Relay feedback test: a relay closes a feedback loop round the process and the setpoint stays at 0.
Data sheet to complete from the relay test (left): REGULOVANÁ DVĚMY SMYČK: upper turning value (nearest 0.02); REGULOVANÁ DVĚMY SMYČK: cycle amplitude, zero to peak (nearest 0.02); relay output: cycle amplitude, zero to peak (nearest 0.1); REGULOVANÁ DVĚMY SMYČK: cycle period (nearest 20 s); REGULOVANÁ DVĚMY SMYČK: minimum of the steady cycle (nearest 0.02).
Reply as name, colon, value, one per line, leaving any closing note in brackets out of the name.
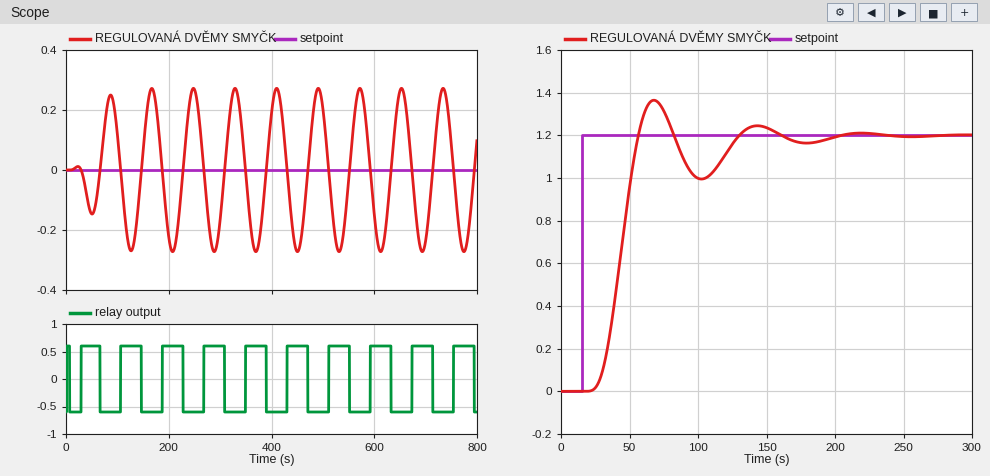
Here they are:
REGULOVANÁ DVĚMY SMYČK: upper turning value: 0.28
REGULOVANÁ DVĚMY SMYČK: cycle amplitude, zero to peak: 0.28
relay output: cycle amplitude, zero to peak: 0.6
REGULOVANÁ DVĚMY SMYČK: cycle period: 80 s
REGULOVANÁ DVĚMY SMYČK: minimum of the steady cycle: -0.28
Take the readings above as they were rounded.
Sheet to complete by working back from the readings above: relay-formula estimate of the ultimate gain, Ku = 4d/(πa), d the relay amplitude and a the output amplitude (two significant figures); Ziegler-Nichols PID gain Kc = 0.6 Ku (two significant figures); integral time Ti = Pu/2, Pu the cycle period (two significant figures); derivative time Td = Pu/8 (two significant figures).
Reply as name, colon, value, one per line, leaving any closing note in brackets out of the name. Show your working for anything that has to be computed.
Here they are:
relay-formula estimate of the ultimate gain, Ku = 4d/(πa), d the relay amplitude and a the output amplitude: 4 × 0.6 / (π × 0.28) = 2.7
Ziegler-Nichols PID gain Kc = 0.6 Ku: 0.6 × 2.7 = 1.6
integral time Ti = Pu/2, Pu the cycle period: 80 / 2 = 40 s
derivative time Td = Pu/8: 80 / 8 = 10 s
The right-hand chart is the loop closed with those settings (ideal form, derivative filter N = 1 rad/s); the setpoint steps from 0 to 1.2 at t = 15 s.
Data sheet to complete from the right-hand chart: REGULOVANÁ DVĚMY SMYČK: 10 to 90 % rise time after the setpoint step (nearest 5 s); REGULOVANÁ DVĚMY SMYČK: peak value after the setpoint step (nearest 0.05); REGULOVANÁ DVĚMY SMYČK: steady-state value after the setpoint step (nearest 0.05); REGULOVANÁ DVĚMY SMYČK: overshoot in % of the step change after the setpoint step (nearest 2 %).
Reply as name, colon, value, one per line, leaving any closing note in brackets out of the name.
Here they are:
REGULOVANÁ DVĚMY SMYČK: 10 to 90 % rise time after the setpoint step: 20 s
REGULOVANÁ DVĚMY SMYČK: peak value after the setpoint step: 1.35
REGULOVANÁ DVĚMY SMYČK: steady-state value after the setpoint step: 1.20
REGULOVANÁ DVĚMY SMYČK: overshoot in % of the step change after the setpoint step: 14 %
